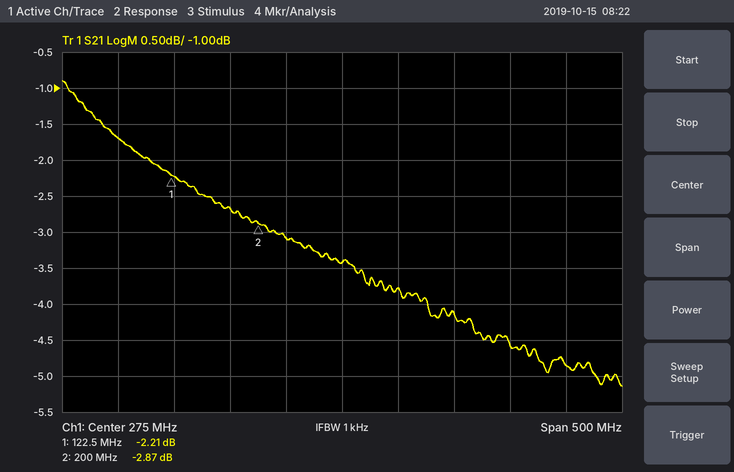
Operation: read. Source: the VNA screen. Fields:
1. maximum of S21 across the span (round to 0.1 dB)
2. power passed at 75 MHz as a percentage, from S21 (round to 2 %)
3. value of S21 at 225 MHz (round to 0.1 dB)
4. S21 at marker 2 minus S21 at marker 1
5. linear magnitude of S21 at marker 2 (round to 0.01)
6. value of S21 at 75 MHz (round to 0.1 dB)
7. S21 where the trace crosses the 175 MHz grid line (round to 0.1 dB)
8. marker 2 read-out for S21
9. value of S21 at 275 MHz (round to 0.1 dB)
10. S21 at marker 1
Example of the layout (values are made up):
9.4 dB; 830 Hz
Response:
-0.9 dB; 68 %; -3.1 dB; -0.66 dB; 0.72; -1.7 dB; -2.7 dB; -2.87 dB; -3.4 dB; -2.21 dB
